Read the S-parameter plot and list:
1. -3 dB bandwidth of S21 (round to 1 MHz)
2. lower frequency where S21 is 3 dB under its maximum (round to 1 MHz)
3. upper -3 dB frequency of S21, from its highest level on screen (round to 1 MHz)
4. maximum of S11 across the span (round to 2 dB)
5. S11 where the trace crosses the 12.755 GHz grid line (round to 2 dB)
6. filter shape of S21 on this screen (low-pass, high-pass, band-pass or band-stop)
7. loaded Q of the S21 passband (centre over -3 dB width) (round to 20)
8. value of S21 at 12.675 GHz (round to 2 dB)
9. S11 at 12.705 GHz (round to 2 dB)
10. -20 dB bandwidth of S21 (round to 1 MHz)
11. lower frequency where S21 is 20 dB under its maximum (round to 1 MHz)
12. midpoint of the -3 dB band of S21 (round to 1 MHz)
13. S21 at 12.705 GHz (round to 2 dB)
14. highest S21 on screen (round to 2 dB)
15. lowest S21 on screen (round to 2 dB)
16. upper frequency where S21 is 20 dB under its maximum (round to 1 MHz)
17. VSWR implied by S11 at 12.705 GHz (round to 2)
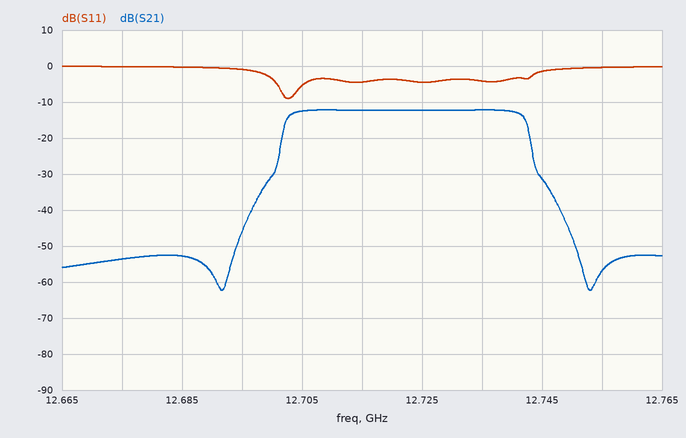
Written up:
40 MHz
12.702 GHz
12.742 GHz
0 dB
0 dB
band-pass
320
-54 dB
-6 dB
46 MHz
12.699 GHz
12.722 GHz
-12 dB
-12 dB
-62 dB
12.745 GHz
4
